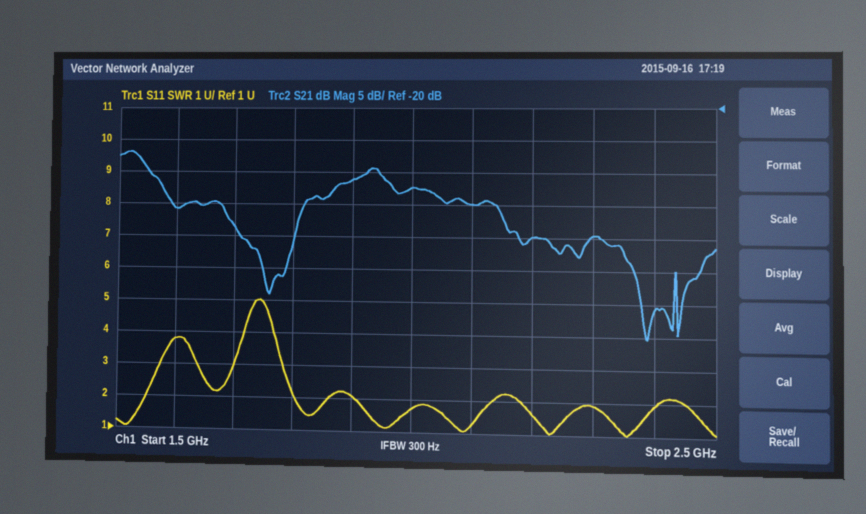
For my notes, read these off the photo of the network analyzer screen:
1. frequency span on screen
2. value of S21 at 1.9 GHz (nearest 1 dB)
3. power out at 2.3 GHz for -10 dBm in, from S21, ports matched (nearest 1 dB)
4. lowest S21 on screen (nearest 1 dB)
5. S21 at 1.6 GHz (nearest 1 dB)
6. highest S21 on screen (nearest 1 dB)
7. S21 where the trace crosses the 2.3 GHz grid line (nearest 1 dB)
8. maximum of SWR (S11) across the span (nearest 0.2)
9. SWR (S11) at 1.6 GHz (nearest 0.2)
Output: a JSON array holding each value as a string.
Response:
["1 GHz", "-31 dB", "-50 dBm", "-55 dB", "-36 dB", "-27 dB", "-40 dB", "5.0", "3.8"]
